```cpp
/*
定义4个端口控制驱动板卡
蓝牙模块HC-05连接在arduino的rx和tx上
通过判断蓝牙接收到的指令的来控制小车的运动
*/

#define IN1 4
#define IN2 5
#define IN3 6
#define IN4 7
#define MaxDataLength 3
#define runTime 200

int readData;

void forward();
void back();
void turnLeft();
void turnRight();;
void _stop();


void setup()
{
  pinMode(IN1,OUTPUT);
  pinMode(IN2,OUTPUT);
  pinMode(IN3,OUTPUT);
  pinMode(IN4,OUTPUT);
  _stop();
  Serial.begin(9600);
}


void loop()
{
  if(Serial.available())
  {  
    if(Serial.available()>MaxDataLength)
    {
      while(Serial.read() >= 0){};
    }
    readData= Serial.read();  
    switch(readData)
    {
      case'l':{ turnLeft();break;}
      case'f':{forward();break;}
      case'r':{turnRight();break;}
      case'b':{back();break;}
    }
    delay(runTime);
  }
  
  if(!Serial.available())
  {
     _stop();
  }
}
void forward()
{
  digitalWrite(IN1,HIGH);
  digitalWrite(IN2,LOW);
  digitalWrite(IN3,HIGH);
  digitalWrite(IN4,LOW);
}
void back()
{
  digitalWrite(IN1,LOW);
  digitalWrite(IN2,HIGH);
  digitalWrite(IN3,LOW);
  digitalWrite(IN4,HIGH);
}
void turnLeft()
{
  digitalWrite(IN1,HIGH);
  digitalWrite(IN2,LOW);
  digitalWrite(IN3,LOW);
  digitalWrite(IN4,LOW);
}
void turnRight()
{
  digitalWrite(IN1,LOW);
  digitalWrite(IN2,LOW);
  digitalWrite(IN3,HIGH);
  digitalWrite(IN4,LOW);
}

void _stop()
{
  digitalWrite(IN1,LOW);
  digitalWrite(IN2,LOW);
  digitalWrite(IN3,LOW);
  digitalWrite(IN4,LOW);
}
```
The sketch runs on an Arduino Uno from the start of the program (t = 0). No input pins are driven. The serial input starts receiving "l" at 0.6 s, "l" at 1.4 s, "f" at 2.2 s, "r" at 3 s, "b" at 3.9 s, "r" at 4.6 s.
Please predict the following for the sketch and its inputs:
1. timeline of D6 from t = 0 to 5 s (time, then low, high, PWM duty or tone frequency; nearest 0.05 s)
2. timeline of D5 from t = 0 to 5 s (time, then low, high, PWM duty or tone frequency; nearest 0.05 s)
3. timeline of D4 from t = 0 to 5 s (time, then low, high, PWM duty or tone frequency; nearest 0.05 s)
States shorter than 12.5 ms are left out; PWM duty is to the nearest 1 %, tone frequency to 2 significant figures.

0 s low; 2.2 s high; 2.4 s low; 3 s high; 3.2 s low; 4.6 s high; 4.8 s low
0 s low; 3.9 s high; 4.1 s low
0 s low; 0.6 s high; 0.8 s low; 1.4 s high; 1.6 s low; 2.2 s high; 2.4 s low
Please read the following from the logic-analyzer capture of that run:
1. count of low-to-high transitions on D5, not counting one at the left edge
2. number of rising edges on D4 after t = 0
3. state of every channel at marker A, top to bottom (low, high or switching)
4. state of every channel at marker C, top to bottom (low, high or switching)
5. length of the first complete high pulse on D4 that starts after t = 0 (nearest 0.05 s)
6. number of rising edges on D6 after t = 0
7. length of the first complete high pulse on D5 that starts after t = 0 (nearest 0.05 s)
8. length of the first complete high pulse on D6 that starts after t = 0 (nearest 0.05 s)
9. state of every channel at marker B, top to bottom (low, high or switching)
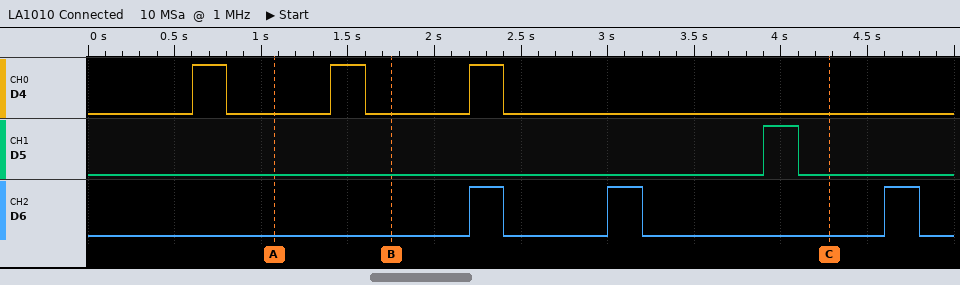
1
3
D4 low, D5 low, D6 low
D4 low, D5 low, D6 low
0.20 s
3
0.20 s
0.20 s
D4 low, D5 low, D6 low
